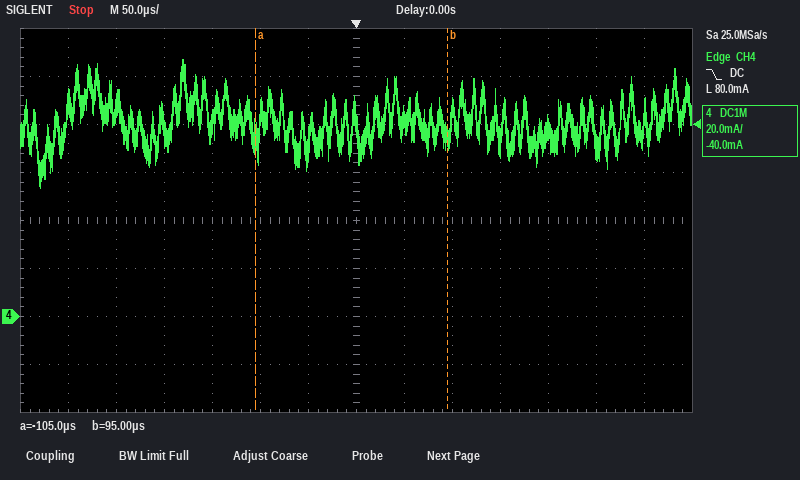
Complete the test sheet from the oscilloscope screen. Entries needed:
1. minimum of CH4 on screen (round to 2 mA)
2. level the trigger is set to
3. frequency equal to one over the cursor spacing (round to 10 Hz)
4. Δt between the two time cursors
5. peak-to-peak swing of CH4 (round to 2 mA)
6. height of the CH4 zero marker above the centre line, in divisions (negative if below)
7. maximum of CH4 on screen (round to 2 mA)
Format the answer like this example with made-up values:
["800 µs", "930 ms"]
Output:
["54 mA", "80.0 mA", "5.00 kHz", "200 µs", "54 mA", "-2.0 div", "108 mA"]
